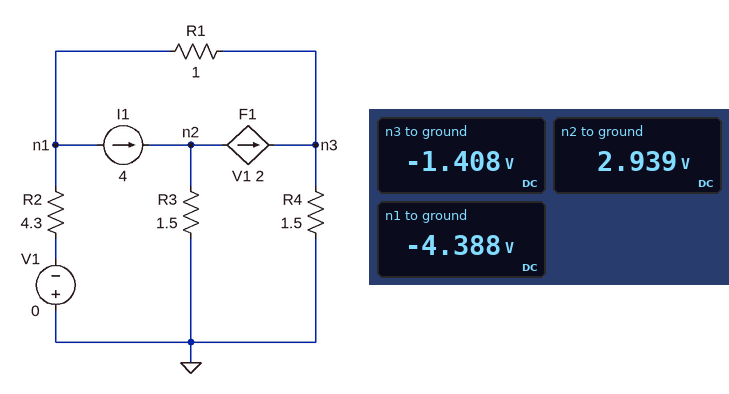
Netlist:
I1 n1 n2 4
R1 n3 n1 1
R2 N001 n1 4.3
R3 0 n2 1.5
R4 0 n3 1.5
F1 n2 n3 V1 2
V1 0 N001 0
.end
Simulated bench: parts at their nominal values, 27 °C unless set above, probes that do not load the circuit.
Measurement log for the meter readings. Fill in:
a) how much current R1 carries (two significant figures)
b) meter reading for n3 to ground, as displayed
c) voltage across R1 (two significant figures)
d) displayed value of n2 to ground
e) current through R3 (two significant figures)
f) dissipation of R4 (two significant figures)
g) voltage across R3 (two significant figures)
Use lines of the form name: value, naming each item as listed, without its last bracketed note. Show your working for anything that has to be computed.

how much current R1 carries: (-1.408 V - (-4.388 V)) / 1 Ω = 3.0 A
meter reading for n3 to ground, as displayed: -1.408 V
voltage across R1: -1.408 V - (-4.388 V) = 3.0 V
displayed value of n2 to ground: 2.939 V
current through R3: (2.939 V) / 1.5 Ω = 2.0 A
dissipation of R4: (0 V - (-1.408 V))^2 / 1.5 Ω = 1.3 W
voltage across R3: 2.939 V = 2.9 V
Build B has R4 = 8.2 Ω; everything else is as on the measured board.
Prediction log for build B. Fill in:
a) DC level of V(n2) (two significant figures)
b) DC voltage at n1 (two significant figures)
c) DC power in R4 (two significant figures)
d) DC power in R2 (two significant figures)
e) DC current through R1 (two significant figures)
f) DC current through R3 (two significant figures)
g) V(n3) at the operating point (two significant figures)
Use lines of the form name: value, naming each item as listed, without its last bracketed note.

DC level of V(n2): 2.3 V
DC voltage at n1: -5.3 V
DC power in R4: 780 mW
DC power in R2: 6.5 W
DC current through R1: 2.8 A
DC current through R3: 1.5 A
V(n3) at the operating point: -2.5 V
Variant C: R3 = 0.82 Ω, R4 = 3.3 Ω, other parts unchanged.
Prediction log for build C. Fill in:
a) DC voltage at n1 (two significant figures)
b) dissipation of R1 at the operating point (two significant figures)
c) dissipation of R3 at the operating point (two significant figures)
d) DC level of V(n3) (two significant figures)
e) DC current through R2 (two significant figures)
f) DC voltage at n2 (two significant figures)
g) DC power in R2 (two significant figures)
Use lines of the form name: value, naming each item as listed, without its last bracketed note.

DC voltage at n1: -4.9 V
dissipation of R1 at the operating point: 8.2 W
dissipation of R3 at the operating point: 2.5 W
DC level of V(n3): -2.0 V
DC current through R2: 1.1 A
DC voltage at n2: 1.4 V
DC power in R2: 5.5 W
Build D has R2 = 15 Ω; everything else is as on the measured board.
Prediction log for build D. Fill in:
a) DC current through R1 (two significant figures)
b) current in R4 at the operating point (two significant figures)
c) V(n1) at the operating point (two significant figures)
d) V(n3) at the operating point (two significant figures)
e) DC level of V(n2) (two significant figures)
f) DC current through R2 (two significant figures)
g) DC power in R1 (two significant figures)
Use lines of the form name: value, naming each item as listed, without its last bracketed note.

DC current through R1: 3.5 A
current in R4 at the operating point: 2.5 A
V(n1) at the operating point: -7.3 V
V(n3) at the operating point: -3.8 V
DC level of V(n2): 4.5 V
DC current through R2: 490 mA
DC power in R1: 12 W
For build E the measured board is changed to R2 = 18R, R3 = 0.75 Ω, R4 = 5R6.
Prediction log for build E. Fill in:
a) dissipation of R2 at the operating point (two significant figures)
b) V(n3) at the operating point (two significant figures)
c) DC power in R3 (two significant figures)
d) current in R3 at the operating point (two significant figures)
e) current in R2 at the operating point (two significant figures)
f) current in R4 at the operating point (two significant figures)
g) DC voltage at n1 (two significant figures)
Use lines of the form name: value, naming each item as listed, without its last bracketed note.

dissipation of R2 at the operating point: 9.8 W
V(n3) at the operating point: -10 V
DC power in R3: 4.8 W
current in R3 at the operating point: 2.5 A
current in R2 at the operating point: 740 mA
current in R4 at the operating point: 1.8 A
DC voltage at n1: -13 V
